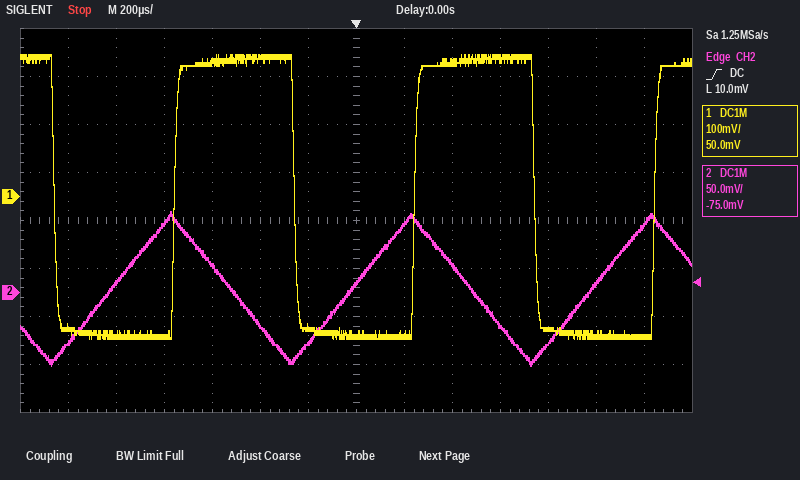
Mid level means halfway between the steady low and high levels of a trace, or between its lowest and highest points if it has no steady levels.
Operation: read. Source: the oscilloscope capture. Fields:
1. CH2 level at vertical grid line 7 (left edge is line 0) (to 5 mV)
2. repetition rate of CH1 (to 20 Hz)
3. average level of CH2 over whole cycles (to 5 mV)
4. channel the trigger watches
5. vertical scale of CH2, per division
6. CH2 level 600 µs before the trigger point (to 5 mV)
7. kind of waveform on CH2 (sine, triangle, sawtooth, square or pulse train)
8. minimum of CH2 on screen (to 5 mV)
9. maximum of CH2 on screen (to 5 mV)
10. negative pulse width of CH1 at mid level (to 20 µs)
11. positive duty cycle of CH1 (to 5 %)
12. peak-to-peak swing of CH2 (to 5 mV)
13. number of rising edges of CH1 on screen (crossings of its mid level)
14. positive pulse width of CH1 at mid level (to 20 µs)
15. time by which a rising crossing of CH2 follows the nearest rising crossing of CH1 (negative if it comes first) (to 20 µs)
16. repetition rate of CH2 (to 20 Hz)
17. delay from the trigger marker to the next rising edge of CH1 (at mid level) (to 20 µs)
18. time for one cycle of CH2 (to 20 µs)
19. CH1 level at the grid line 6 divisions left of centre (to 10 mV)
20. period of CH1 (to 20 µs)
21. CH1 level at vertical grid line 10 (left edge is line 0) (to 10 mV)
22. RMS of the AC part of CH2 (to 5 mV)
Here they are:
10 mV
1.00 kHz
5 mV
CH2
50 mV
30 mV
triangle
-75 mV
85 mV
500 µs
50 %
160 mV
3
500 µs
-260 µs
1.00 kHz
240 µs
1.00 ms
-270 mV
1.00 ms
290 mV
45 mV
